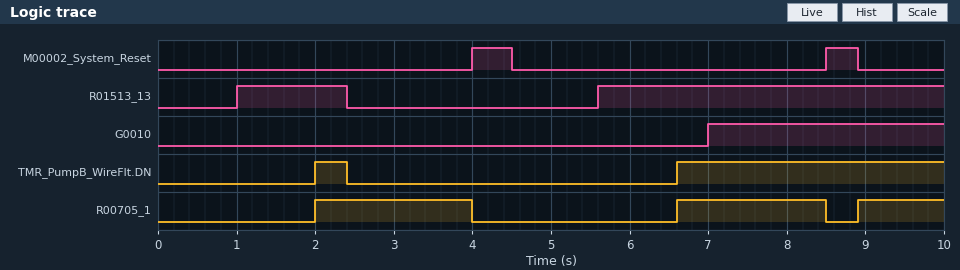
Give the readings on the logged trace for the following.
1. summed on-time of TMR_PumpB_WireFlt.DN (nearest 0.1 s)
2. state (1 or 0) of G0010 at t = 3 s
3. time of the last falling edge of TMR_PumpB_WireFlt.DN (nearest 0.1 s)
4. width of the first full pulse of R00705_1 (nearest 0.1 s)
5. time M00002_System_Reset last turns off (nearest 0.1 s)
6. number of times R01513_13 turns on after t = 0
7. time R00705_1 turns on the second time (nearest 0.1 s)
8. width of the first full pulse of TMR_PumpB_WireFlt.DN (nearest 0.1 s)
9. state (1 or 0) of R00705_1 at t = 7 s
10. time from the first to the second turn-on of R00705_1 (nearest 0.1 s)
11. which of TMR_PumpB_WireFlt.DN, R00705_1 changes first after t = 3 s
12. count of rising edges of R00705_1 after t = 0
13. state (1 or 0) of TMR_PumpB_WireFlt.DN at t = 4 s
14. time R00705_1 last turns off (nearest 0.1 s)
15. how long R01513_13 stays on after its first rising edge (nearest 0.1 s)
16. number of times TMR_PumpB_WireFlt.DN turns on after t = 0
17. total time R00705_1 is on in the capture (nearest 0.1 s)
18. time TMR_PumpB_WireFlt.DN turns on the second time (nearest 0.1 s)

3.8 s
0
2.4 s
2.0 s
8.9 s
2
6.6 s
0.4 s
1
4.6 s
R00705_1
3
0
8.5 s
1.4 s
2
5.0 s
6.6 s
